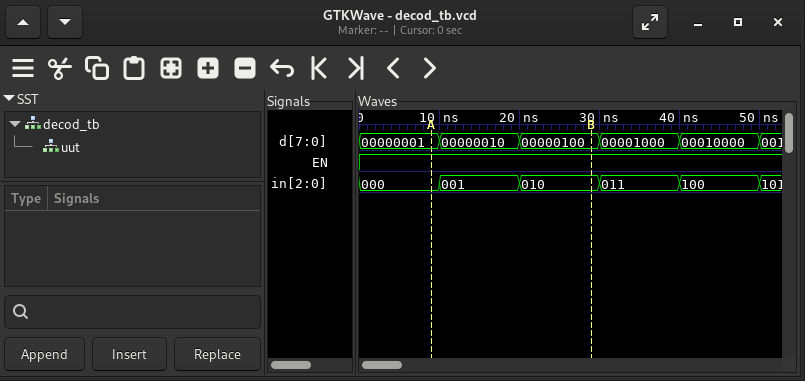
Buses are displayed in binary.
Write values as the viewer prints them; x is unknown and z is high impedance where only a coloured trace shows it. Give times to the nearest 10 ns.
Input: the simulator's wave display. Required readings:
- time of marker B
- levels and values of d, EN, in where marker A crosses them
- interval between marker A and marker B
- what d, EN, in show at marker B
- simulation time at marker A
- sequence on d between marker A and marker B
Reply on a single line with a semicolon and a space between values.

30 ns; d=00000001, EN=1, in=000; 20 ns; d=00000100, EN=1, in=010; 10 ns; 00000001, 00000010, 00000100
